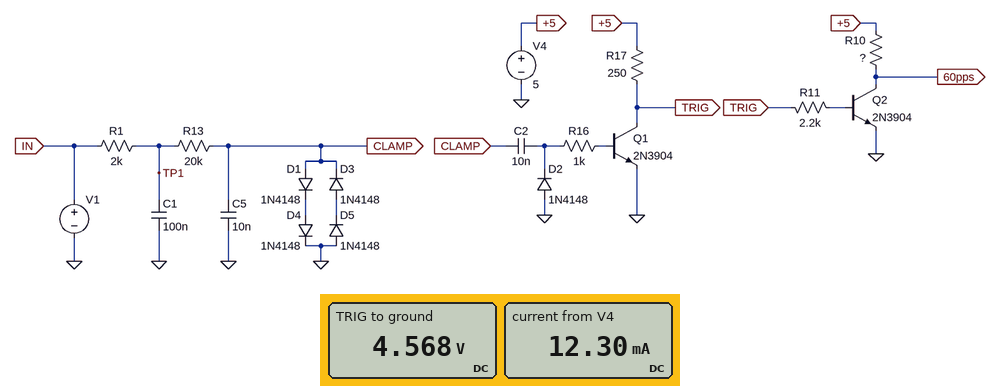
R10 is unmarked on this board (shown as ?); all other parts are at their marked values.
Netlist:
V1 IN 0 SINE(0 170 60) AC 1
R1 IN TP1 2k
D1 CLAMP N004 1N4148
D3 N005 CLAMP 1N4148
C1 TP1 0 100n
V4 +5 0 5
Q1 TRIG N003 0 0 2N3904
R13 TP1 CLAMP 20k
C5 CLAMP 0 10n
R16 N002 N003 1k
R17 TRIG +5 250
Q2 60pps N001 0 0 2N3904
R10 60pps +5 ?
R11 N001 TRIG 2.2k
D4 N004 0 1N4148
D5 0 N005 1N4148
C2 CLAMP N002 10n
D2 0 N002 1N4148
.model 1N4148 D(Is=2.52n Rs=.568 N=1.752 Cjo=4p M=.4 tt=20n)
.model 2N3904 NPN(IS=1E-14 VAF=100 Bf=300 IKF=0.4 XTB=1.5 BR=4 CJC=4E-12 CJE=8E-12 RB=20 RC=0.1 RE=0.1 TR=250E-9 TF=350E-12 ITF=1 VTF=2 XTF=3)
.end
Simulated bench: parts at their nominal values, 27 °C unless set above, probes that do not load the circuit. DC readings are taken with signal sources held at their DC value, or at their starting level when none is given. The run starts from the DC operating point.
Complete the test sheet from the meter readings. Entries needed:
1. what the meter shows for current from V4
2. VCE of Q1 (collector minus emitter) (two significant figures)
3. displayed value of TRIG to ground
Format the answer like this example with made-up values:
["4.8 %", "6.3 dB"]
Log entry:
["12.30 mA", "4.6 V", "4.568 V"]
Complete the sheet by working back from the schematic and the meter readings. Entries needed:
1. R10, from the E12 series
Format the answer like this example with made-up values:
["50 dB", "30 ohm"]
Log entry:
["470 Ω"]
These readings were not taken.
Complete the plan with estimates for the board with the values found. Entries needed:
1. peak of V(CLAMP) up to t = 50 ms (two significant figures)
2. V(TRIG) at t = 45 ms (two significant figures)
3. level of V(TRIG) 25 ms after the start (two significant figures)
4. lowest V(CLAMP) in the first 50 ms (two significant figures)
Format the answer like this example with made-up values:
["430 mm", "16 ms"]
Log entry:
["1.4 V", "4.6 V", "4.6 V", "-1.4 V"]
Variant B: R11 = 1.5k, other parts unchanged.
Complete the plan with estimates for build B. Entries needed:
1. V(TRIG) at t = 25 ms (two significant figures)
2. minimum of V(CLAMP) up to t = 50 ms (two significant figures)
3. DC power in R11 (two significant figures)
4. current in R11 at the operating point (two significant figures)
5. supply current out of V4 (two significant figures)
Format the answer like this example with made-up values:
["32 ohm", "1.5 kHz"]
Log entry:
["4.4 V", "-1.4 V", "8.7 mW", "2.4 mA", "13 mA"]
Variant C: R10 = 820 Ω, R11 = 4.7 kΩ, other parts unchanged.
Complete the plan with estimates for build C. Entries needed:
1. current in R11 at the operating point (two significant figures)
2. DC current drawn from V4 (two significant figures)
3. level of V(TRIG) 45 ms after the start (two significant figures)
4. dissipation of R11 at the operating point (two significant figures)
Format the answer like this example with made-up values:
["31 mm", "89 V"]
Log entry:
["860 µA", "6.9 mA", "4.8 V", "3.5 mW"]
